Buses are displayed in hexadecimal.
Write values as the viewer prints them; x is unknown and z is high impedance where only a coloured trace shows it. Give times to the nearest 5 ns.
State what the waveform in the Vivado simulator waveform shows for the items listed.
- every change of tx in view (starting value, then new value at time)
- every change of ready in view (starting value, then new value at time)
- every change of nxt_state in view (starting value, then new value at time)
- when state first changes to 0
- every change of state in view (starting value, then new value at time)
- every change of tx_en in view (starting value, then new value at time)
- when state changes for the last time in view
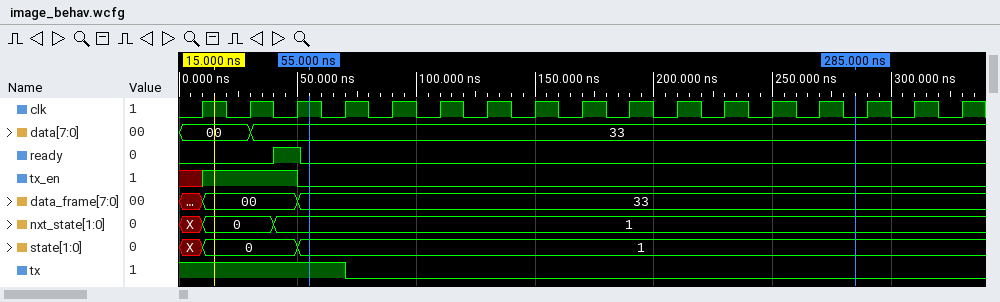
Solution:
1, 0 at 70 ns
0, 1 at 40 ns, 0 at 50 ns
X, 0 at 10 ns, 1 at 40 ns
10 ns
X, 0 at 10 ns, 1 at 50 ns
x, 1 at 10 ns, 0 at 50 ns
50 ns
